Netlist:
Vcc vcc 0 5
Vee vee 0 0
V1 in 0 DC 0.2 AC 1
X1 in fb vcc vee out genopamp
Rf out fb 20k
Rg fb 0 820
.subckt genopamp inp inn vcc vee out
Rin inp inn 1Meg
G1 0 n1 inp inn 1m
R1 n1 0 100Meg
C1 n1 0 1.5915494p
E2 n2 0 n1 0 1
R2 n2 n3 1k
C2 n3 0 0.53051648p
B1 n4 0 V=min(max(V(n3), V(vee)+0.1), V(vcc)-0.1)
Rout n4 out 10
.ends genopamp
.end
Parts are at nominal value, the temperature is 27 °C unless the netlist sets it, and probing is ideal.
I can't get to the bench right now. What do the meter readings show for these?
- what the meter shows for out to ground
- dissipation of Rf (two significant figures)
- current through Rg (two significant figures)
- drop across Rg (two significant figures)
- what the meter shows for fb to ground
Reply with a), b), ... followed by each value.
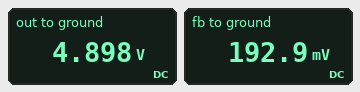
a) 4.898 V
b) 1.1 mW
c) 240 µA
d) 190 mV
e) 192.9 mV
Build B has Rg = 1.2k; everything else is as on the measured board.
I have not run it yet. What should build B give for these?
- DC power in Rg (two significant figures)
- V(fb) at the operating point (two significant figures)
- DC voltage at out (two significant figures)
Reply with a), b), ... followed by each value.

a) 33 µW
b) 200 mV
c) 3.5 V
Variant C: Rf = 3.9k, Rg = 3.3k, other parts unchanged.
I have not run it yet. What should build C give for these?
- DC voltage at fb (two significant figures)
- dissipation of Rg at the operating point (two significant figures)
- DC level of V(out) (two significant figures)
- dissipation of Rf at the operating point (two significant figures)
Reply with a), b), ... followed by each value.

a) 200 mV
b) 12 µW
c) 440 mV
d) 14 µW
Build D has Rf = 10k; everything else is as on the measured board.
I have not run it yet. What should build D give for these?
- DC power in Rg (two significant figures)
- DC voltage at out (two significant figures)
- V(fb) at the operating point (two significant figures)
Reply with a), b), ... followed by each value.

a) 49 µW
b) 2.6 V
c) 200 mV
